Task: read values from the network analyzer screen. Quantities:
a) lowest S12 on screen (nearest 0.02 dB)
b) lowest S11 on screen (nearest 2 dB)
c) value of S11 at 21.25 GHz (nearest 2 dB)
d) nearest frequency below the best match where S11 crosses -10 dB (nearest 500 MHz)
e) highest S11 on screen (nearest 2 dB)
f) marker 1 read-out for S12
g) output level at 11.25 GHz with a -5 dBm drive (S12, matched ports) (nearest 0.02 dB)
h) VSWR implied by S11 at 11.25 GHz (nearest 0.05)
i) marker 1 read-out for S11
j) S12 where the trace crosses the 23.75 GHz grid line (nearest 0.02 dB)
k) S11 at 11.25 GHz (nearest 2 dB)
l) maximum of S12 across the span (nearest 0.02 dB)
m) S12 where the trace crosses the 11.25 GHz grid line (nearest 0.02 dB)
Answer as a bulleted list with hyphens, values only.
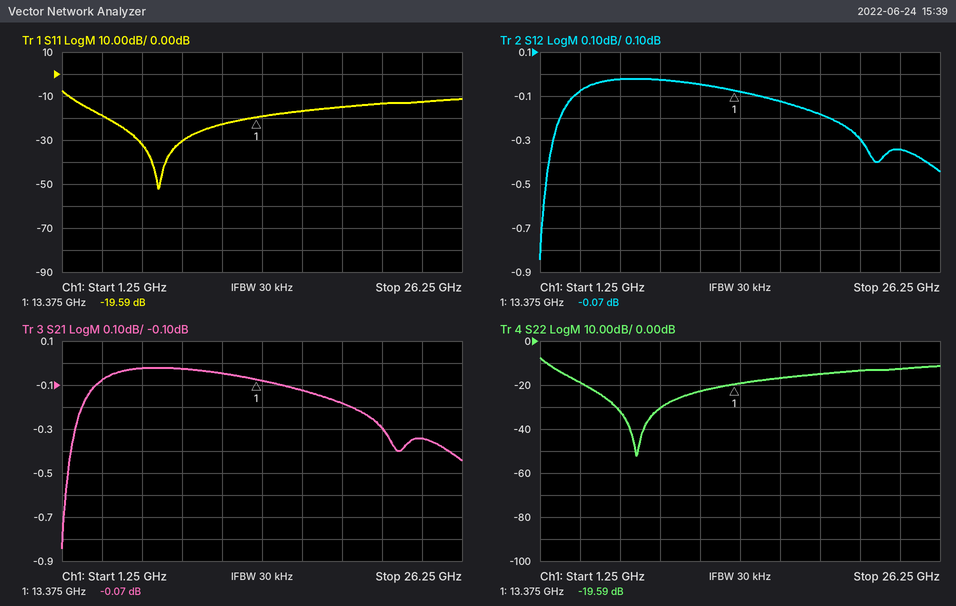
- -0.84 dB
- -52 dB
- -14 dB
- 1.5 GHz
- -8 dB
- -0.07 dB
- -5.04 dBm
- 1.15
- -19.59 dB
- -0.34 dB
- -22 dB
- -0.02 dB
- -0.04 dB
